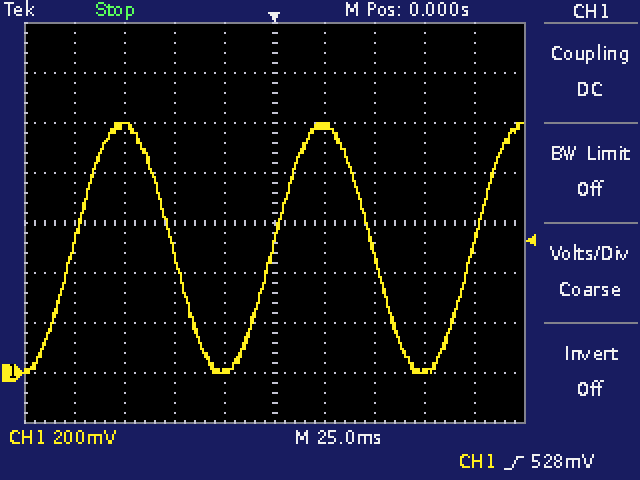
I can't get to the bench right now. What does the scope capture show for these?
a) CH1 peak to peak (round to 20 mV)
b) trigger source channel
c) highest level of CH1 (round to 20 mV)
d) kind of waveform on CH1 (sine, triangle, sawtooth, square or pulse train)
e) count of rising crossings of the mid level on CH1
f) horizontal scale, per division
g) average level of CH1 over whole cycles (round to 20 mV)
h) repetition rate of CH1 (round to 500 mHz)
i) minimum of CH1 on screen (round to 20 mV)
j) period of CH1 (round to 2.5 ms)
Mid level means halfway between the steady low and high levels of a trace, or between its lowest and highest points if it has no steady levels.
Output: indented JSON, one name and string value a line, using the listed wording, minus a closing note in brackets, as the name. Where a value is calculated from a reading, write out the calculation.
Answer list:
{
  "CH1 peak to peak": "1.00 V − (0 mV) = 1.00 V",
  "trigger source channel": "CH1",
  "highest level of CH1": "1.00 V",
  "kind of waveform on CH1": "sine",
  "count of rising crossings of the mid level on CH1": "3",
  "horizontal scale, per division": "25 ms",
  "average level of CH1 over whole cycles": "(1.00 V + (0 mV)) / 2 ≈ 500 mV",
  "repetition rate of CH1": "1 / 100.0 ms ≈ 10.0 Hz",
  "minimum of CH1 on screen": "0 mV",
  "period of CH1": "100.0 ms"
}
